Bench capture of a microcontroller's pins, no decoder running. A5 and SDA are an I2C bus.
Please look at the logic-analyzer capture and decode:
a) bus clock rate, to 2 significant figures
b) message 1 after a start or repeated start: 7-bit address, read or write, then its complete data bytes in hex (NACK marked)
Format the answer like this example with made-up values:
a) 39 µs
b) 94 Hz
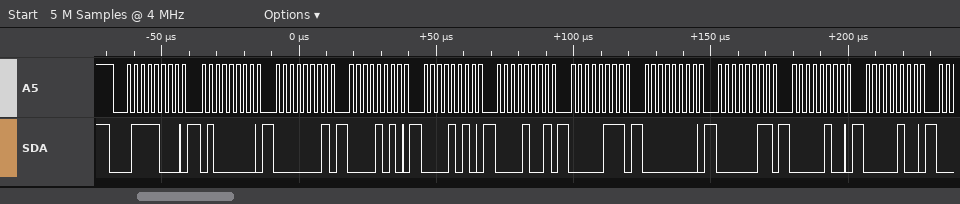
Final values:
a) 400 kHz
b) 0x3C write: 40 01 0A 0A 09 07 00 03 04 04
